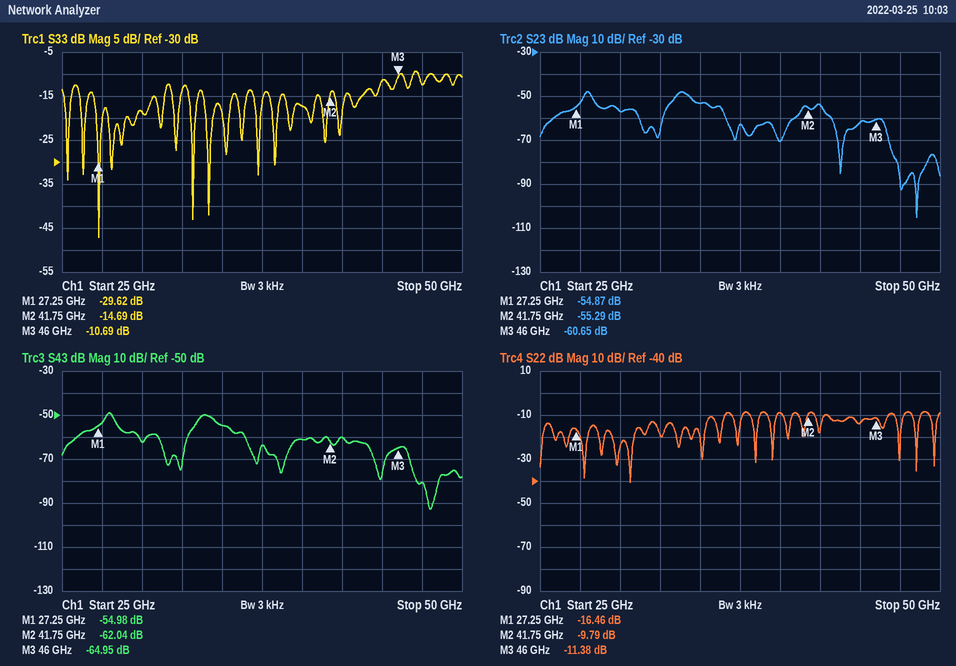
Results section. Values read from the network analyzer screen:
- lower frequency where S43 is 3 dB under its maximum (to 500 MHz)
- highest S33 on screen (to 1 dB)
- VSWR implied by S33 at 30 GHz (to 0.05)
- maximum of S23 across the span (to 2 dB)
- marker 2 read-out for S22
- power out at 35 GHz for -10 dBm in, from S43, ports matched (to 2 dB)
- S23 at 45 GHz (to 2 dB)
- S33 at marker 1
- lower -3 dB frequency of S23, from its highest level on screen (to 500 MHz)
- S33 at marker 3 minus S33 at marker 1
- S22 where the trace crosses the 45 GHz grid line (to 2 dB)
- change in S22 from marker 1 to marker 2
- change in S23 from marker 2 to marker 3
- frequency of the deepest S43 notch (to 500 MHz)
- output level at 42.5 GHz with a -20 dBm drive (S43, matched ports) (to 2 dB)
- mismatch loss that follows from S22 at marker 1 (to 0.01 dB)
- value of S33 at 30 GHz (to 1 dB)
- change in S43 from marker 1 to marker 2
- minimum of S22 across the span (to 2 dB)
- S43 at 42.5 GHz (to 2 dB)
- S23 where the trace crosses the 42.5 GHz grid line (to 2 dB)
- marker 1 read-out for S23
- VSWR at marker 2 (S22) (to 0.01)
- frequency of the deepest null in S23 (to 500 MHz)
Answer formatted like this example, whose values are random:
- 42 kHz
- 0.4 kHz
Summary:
- 27.5 GHz
- -9 dB
- 1.25
- -48 dB
- -9.79 dB
- -64 dBm
- -62 dB
- -29.62 dB
- 27.5 GHz
- 18.93 dB
- -14 dB
- 6.67 dB
- -5.36 dB
- 48.0 GHz
- -80 dBm
- 0.10 dB
- -19 dB
- -7.06 dB
- -40 dB
- -60 dB
- -54 dB
- -54.87 dB
- 1.96
- 48.5 GHz
